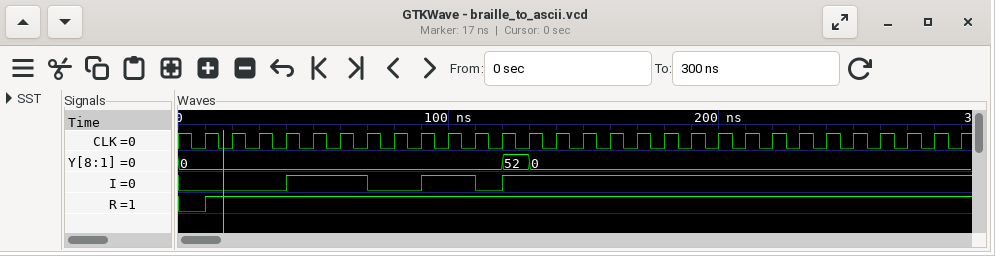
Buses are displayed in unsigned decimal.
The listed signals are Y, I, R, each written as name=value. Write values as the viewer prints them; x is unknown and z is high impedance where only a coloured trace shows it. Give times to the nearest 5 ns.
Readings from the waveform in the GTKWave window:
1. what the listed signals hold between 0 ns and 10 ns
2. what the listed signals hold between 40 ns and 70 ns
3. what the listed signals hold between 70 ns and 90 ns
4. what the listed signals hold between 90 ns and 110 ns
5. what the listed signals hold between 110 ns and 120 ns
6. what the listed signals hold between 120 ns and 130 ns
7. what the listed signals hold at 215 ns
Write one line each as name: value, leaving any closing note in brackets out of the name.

what the listed signals hold between 0 ns and 10 ns: Y=0, I=0, R=0
what the listed signals hold between 40 ns and 70 ns: Y=0, I=1, R=1
what the listed signals hold between 70 ns and 90 ns: Y=0, I=0, R=1
what the listed signals hold between 90 ns and 110 ns: Y=0, I=1, R=1
what the listed signals hold between 110 ns and 120 ns: Y=0, I=0, R=1
what the listed signals hold between 120 ns and 130 ns: Y=52, I=1, R=1
what the listed signals hold at 215 ns: Y=0, I=1, R=1
